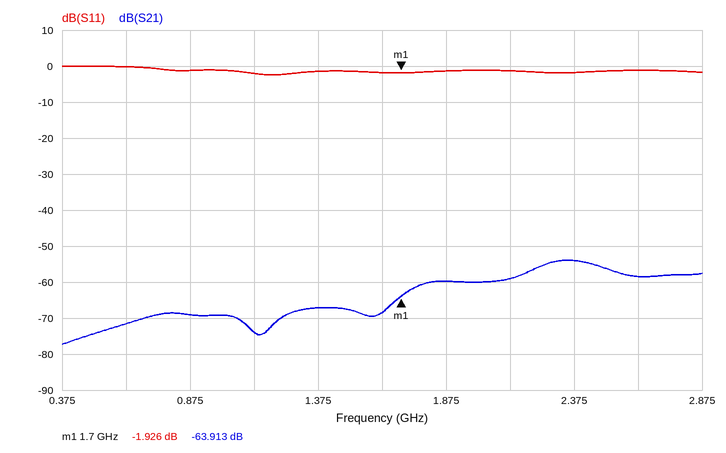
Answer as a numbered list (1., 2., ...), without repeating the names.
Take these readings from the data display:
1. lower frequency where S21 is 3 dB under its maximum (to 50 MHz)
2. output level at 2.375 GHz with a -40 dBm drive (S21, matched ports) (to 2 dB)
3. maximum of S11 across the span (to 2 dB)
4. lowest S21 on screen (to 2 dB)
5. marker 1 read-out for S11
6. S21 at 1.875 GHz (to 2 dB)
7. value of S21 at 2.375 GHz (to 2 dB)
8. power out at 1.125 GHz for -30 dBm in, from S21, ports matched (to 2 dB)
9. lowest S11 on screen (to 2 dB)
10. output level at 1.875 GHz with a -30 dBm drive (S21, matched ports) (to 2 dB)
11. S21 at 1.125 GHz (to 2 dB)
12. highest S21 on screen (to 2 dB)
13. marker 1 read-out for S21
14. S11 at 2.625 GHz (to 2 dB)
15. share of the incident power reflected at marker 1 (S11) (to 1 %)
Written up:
1. 2.20 GHz
2. -94 dBm
3. 0 dB
4. -78 dB
5. -1.926 dB
6. -60 dB
7. -54 dB
8. -104 dBm
9. -2 dB
10. -90 dBm
11. -74 dB
12. -54 dB
13. -63.913 dB
14. -2 dB
15. 64 %
